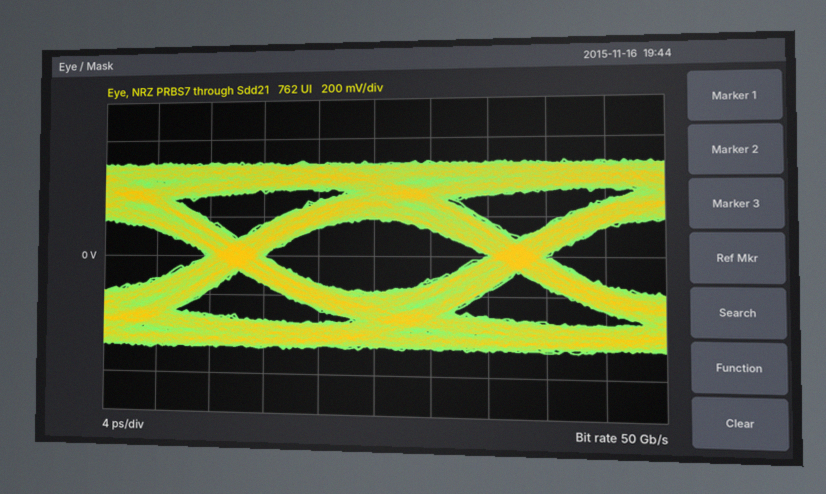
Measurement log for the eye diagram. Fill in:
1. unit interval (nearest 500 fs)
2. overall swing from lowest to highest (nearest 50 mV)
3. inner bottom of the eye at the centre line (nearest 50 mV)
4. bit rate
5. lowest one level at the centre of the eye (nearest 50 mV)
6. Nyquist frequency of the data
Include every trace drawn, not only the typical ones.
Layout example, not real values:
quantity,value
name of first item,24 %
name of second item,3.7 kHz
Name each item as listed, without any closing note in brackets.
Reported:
quantity,value
unit interval,20.0 ps
overall swing from lowest to highest,950 mV
inner bottom of the eye at the centre line,-200 mV
bit rate,50 Gb/s
lowest one level at the centre of the eye,200 mV
Nyquist frequency of the data,25 GHz
